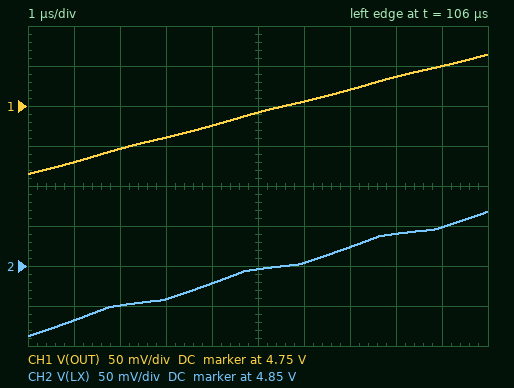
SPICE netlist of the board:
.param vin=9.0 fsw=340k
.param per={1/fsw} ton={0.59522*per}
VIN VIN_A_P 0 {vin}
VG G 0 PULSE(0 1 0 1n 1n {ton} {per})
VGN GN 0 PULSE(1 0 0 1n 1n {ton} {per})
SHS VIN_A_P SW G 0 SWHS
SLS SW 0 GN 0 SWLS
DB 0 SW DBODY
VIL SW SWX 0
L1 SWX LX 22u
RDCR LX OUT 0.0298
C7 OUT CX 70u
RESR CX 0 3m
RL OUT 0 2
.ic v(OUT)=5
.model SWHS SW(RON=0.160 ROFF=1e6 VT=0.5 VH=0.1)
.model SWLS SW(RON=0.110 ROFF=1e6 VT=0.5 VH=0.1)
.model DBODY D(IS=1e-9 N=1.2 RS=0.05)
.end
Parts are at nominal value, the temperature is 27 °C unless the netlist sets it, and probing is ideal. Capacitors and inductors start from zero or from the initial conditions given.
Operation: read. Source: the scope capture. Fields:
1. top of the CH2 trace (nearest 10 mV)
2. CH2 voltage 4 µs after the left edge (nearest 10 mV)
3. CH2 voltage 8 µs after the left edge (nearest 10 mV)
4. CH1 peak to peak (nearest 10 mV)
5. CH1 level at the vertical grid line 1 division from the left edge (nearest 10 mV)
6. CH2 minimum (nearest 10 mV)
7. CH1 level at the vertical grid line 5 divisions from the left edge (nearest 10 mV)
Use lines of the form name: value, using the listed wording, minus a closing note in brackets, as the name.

top of the CH2 trace: 4.92 V
CH2 voltage 4 µs after the left edge: 4.83 V
CH2 voltage 8 µs after the left edge: 4.89 V
CH1 peak to peak: 150 mV
CH1 level at the vertical grid line 1 division from the left edge: 4.68 V
CH2 minimum: 4.76 V
CH1 level at the vertical grid line 5 divisions from the left edge: 4.74 V
